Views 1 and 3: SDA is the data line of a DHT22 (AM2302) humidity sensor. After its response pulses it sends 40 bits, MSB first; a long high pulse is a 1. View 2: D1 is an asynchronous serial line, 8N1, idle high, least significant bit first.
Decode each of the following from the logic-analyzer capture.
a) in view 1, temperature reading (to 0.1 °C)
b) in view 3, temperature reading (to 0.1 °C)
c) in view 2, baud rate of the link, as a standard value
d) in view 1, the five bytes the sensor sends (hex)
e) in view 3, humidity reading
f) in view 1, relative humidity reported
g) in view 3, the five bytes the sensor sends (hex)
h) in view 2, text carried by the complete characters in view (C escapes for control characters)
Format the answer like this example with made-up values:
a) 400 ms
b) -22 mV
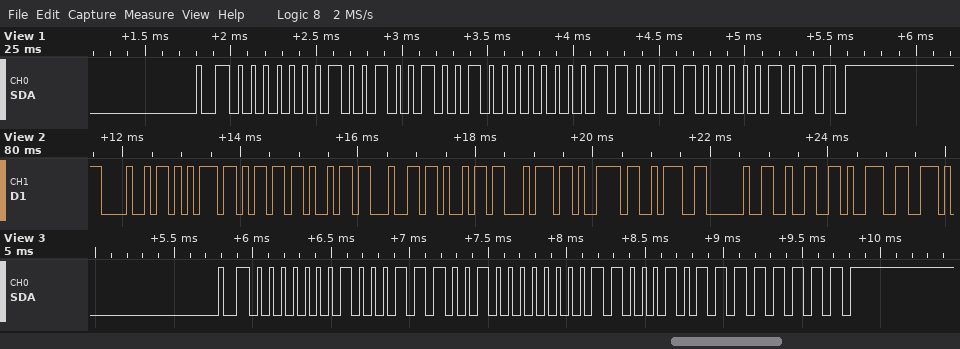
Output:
a) -10.2 °C
b) -9.8 °C
c) 9600 baud
d) 01 24 80 66 0B
e) 28.4 %
f) 29.2 %
g) 01 1C 80 62 FF
h) "Humidity: 29"
